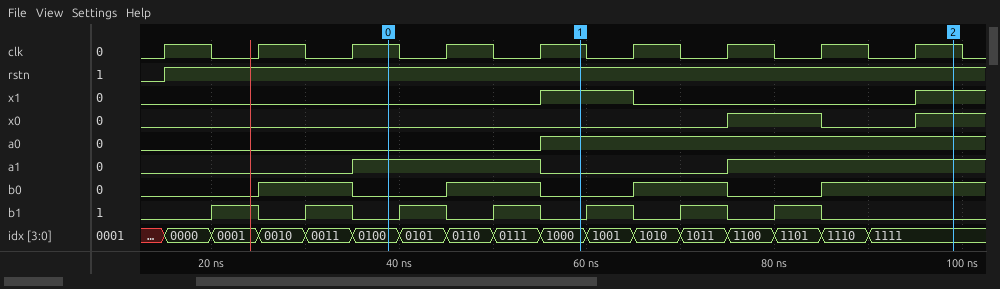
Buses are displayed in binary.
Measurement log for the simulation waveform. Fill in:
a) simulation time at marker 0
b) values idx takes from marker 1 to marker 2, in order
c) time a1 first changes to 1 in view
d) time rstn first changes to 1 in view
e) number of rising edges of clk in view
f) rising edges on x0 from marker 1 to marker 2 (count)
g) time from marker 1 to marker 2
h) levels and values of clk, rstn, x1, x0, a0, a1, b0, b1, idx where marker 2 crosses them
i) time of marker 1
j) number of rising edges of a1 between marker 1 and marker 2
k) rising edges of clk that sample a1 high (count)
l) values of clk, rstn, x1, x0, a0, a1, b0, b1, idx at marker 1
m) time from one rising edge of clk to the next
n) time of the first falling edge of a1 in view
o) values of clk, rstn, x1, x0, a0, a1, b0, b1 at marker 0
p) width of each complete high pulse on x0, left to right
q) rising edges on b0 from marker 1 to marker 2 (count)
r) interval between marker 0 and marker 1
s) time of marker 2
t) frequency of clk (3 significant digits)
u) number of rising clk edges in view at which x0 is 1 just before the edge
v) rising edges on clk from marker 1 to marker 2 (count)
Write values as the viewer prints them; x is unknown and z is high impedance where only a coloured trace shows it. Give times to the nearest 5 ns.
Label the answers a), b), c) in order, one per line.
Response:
a) 40 ns
b) 1000, 1001, 1010, 1011, 1100, 1101, 1110, 1111
c) 35 ns
d) 15 ns
e) 9
f) 2
g) 40 ns
h) clk=1, rstn=1, x1=1, x0=1, a0=1, a1=1, b0=1, b1=0, idx=1111
i) 60 ns
j) 1
k) 4
l) clk=1, rstn=1, x1=1, x0=0, a0=1, a1=0, b0=0, b1=0, idx=1000
m) 10 ns
n) 55 ns
o) clk=1, rstn=1, x1=0, x0=0, a0=0, a1=1, b0=0, b1=0
p) 10 ns
q) 2
r) 20 ns
s) 100 ns
t) 100 MHz
u) 1
v) 4
